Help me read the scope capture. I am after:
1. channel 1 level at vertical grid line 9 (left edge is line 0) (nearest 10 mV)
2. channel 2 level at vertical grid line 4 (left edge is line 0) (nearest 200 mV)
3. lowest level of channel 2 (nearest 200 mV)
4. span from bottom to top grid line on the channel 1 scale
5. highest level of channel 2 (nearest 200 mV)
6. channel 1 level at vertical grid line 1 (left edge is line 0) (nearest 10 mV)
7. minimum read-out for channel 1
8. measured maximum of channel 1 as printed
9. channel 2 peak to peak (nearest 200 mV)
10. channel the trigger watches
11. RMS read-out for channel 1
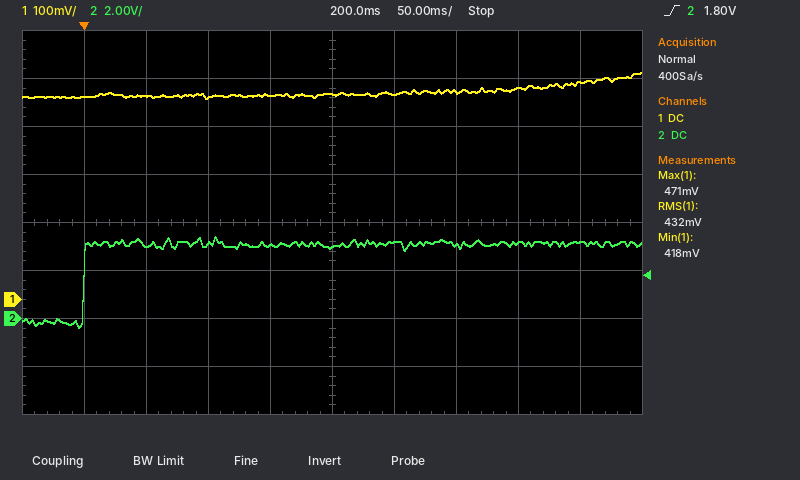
450 mV
3.0 V
-400 mV
800 mV
3.4 V
420 mV
418 mV
471 mV
3.8 V
channel 2
432 mV
